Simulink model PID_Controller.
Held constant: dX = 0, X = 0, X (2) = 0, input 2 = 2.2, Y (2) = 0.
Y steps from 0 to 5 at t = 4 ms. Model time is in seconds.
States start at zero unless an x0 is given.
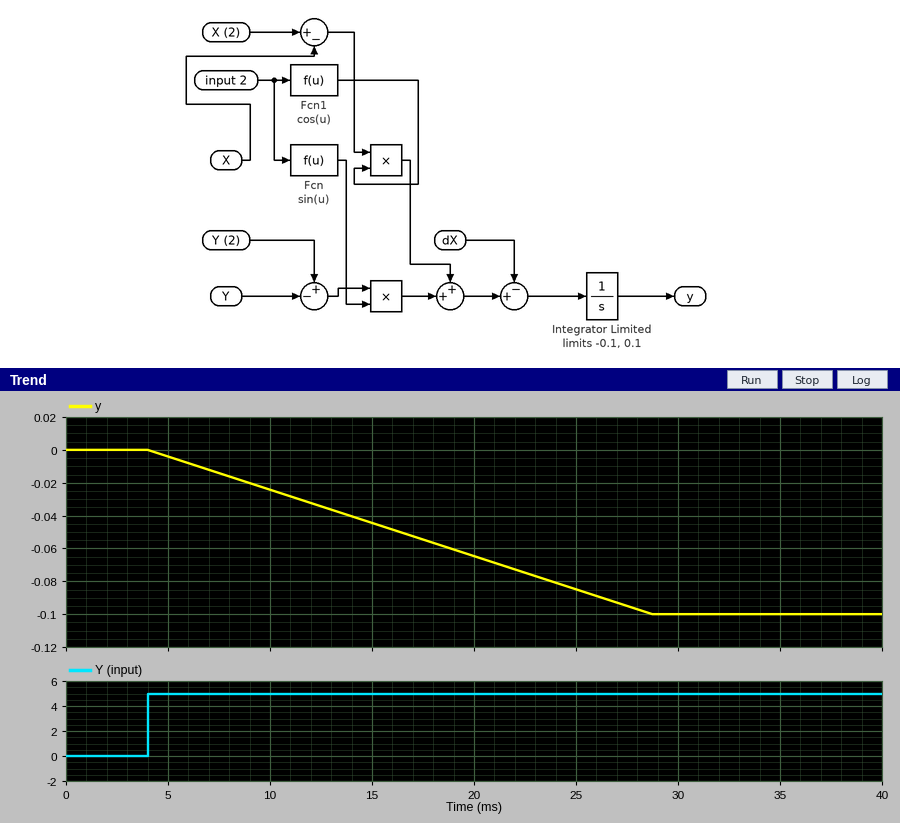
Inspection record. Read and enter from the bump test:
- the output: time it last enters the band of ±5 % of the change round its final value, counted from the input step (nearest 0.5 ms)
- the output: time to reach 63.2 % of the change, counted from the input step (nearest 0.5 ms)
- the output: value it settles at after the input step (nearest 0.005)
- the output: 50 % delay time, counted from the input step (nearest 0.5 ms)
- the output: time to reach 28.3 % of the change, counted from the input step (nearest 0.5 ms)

23.5 ms
15.5 ms
-0.100
12.5 ms
7.0 ms
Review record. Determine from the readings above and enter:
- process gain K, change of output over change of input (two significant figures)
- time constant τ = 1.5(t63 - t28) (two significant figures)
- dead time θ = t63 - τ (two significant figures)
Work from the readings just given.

-0.020
13 ms
2.5 ms
